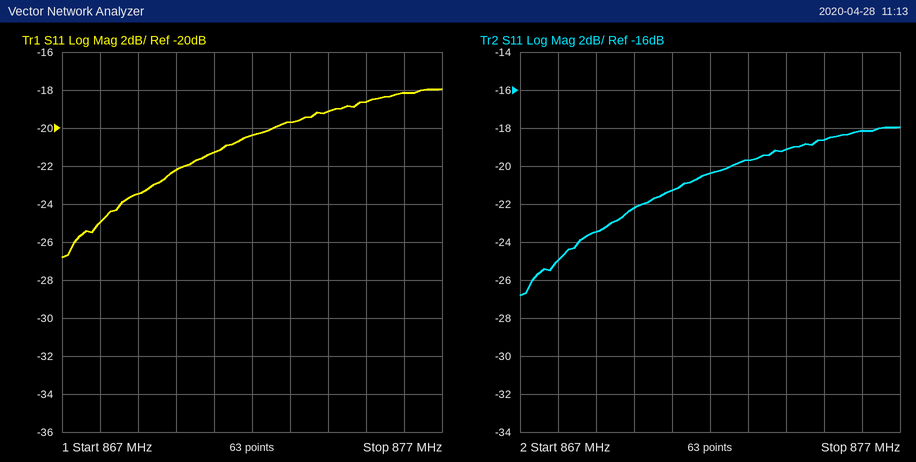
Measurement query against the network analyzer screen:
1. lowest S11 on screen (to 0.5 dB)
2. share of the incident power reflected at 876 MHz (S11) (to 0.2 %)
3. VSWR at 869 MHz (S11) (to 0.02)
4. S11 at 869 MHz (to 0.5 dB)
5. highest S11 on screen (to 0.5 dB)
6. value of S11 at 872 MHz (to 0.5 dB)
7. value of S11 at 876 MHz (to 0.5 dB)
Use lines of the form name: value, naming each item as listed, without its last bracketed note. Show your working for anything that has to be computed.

lowest S11 on screen: -27.0 dB
share of the incident power reflected at 876 MHz (S11): 10^(-18/10) ≈ 1.6 %
VSWR at 869 MHz (S11): |Γ| = 10^(-23.5/20) = 0.0668; VSWR = (1 + 0.0668)/(1 − 0.0668) ≈ 1.14
S11 at 869 MHz: -23.5 dB
highest S11 on screen: -18.0 dB
value of S11 at 872 MHz: -20.5 dB
value of S11 at 876 MHz: -18.0 dB
